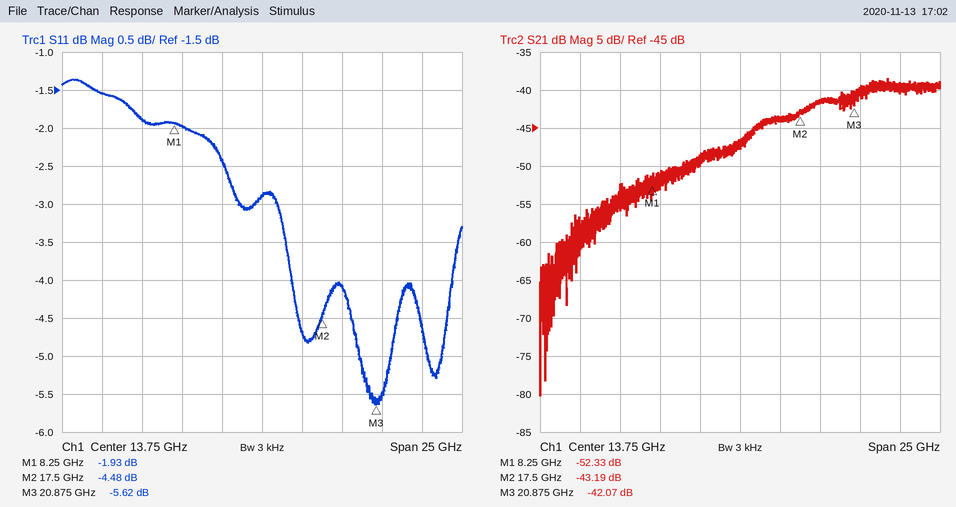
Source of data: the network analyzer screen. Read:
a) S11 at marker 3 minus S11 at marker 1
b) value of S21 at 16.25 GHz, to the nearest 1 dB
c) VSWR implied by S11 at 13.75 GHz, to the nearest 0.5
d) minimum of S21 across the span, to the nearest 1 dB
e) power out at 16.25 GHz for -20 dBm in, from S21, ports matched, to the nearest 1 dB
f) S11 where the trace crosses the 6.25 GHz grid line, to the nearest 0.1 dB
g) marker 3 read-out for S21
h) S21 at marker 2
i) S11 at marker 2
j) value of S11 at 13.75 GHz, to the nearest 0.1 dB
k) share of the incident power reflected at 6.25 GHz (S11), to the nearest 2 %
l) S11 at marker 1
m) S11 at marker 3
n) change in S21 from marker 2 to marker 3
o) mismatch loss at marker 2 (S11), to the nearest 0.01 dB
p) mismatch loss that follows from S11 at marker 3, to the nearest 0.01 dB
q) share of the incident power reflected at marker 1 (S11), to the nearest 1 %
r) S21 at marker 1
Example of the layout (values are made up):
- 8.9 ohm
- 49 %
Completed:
- -3.69 dB
- -44 dB
- 6.0
- -80 dB
- -64 dBm
- -1.9 dB
- -42.07 dB
- -43.19 dB
- -4.48 dB
- -2.9 dB
- 64 %
- -1.93 dB
- -5.62 dB
- 1.12 dB
- 1.91 dB
- 1.39 dB
- 64 %
- -52.33 dB
